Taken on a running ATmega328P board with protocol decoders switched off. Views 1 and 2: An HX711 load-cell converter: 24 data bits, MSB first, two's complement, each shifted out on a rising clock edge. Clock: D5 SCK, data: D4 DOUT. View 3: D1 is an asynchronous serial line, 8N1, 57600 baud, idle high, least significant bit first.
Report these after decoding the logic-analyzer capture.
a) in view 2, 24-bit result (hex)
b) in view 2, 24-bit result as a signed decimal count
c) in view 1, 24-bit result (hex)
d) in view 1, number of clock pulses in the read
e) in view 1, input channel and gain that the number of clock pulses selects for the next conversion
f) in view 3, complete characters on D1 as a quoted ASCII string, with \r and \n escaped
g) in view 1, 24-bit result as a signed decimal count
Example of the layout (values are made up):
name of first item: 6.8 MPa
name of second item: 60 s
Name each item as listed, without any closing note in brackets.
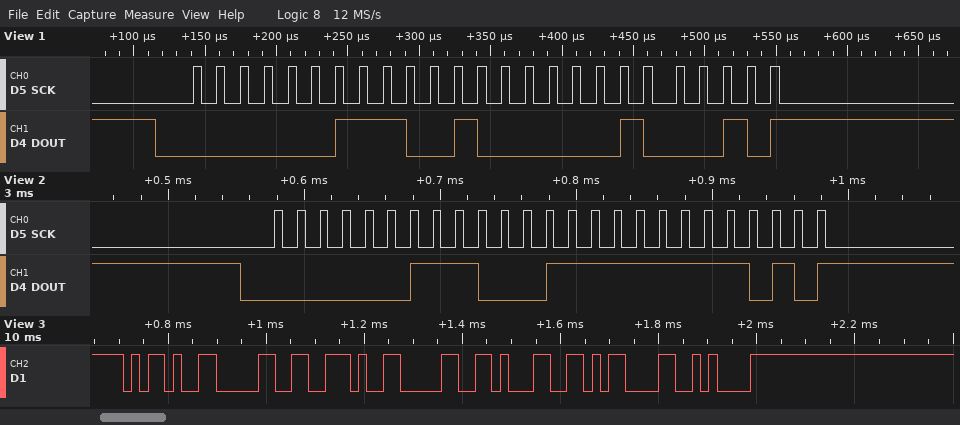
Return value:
in view 2, 24-bit result: 0x038FFA
in view 2, 24-bit result as a signed decimal count: 233466
in view 1, 24-bit result: 0x039022
in view 1, number of clock pulses in the read: 25
in view 1, input channel and gain that the number of clock pulses selects for the next conversion: channel A, gain 128
in view 3, complete characters on D1 as a quoted ASCII string, with \r and \n escaped: "-0.01\r\n"
in view 1, 24-bit result as a signed decimal count: 233506
